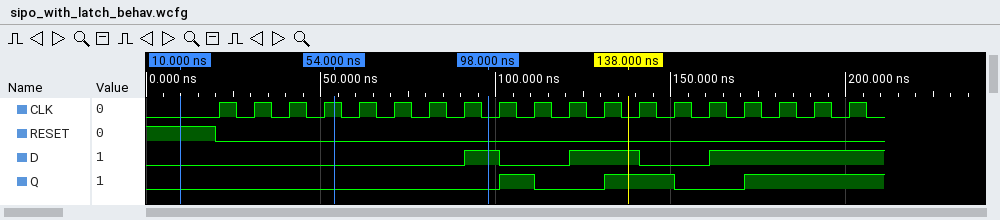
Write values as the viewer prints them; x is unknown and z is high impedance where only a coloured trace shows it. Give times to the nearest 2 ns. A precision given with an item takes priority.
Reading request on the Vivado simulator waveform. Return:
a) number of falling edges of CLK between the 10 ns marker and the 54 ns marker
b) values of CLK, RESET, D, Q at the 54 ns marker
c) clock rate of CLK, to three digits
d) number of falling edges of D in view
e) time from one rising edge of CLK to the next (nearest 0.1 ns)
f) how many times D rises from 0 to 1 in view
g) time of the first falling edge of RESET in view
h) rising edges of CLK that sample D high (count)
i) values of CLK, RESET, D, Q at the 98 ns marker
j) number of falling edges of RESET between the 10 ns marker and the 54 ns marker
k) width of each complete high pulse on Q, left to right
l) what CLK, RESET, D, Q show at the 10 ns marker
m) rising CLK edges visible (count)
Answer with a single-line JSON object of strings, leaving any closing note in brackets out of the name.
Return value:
{"number of falling edges of CLK between the 10 ns marker and the 54 ns marker": "3", "values of CLK, RESET, D, Q at the 54 ns marker": "CLK=1, RESET=0, D=0, Q=0", "clock rate of CLK, to three digits": "100 MHz", "number of falling edges of D in view": "2", "time from one rising edge of CLK to the next": "10 ns", "how many times D rises from 0 to 1 in view": "3", "time of the first falling edge of RESET in view": "20 ns", "rising edges of CLK that sample D high": "7", "values of CLK, RESET, D, Q at the 98 ns marker": "CLK=0, RESET=0, D=1, Q=0", "number of falling edges of RESET between the 10 ns marker and the 54 ns marker": "1", "width of each complete high pulse on Q, left to right": "10 ns, 20 ns", "what CLK, RESET, D, Q show at the 10 ns marker": "CLK=0, RESET=1, D=0, Q=0", "rising CLK edges visible": "19"}
